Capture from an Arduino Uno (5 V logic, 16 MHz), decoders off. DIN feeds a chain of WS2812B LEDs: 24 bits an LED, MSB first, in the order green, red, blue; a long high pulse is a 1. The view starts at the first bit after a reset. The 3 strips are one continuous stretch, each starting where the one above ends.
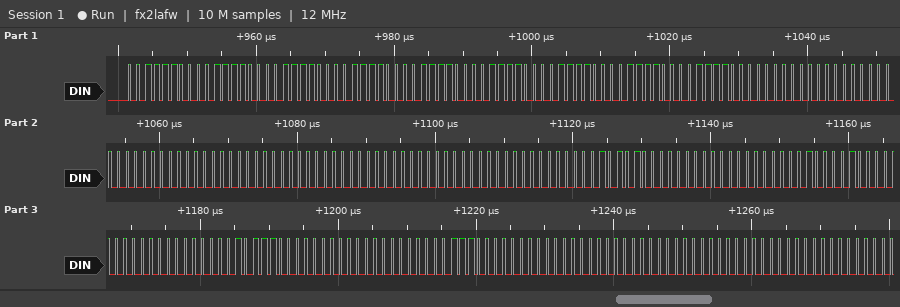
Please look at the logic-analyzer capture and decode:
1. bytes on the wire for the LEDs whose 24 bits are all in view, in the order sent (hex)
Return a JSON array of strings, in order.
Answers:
["3C 3C 3C 3C 3C 3C 3C 3C 3C 00 00 00 00 00 00 00 00 00 2A 00 00 21 00 00 17 00 00 0E 00 00 00 00 00"]
